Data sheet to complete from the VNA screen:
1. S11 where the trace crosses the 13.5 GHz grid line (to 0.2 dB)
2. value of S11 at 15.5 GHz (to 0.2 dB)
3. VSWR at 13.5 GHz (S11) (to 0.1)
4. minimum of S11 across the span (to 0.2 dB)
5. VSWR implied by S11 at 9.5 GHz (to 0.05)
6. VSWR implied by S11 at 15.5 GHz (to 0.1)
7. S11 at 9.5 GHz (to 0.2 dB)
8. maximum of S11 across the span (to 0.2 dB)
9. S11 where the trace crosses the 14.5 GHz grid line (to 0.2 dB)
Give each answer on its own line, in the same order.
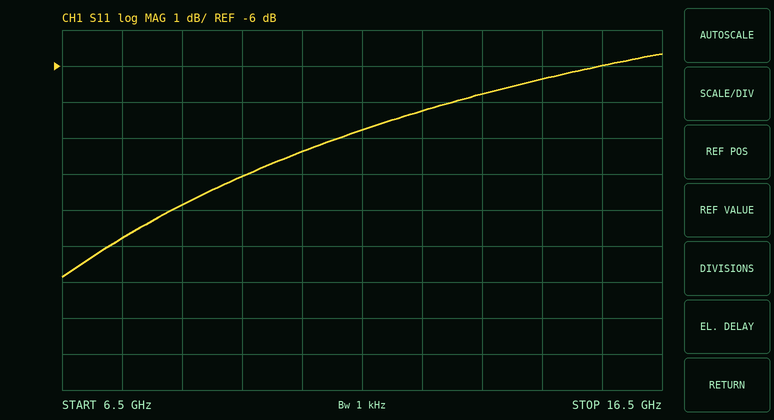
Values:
-6.8 dB
-6.0 dB
2.7
-11.8 dB
2.10
3.0
-9.0 dB
-5.6 dB
-6.4 dB
